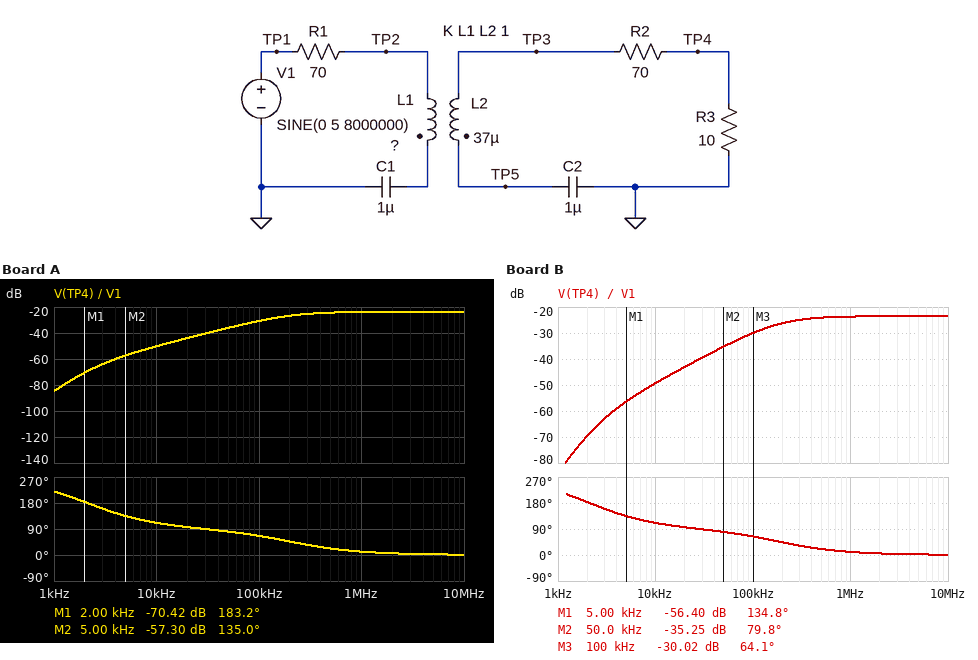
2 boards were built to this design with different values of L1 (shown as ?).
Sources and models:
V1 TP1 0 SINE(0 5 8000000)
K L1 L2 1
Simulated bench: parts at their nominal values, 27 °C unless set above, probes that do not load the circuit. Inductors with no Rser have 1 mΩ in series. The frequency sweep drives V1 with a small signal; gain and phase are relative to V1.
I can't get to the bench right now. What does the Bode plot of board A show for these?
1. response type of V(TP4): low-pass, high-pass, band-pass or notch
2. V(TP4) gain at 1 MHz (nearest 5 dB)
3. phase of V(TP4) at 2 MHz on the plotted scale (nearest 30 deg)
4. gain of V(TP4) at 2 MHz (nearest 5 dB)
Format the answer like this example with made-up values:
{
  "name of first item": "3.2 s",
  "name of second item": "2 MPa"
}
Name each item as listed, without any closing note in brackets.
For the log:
{
  "response type of V(TP4): low-pass, high-pass, band-pass or notch": "high-pass",
  "V(TP4) gain at 1 MHz": "-25 dB",
  "phase of V(TP4) at 2 MHz on the plotted scale": "0 deg",
  "gain of V(TP4) at 2 MHz": "-25 dB"
}
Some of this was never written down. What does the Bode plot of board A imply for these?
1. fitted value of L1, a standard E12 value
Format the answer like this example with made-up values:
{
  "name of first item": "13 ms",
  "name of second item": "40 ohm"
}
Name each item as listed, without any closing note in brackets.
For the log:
{
  "fitted value of L1, a standard E12 value": "22 µH"
}
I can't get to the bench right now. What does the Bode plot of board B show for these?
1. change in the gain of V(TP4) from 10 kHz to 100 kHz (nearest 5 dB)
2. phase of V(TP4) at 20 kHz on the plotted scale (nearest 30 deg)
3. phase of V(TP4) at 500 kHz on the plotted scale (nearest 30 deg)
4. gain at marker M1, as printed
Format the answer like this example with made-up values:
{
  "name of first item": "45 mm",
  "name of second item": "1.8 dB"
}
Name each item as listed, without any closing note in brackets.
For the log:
{
  "change in the gain of V(TP4) from 10 kHz to 100 kHz": "20 dB",
  "phase of V(TP4) at 20 kHz on the plotted scale": "90 deg",
  "phase of V(TP4) at 500 kHz on the plotted scale": "30 deg",
  "gain at marker M1, as printed": "-56.40 dB"
}
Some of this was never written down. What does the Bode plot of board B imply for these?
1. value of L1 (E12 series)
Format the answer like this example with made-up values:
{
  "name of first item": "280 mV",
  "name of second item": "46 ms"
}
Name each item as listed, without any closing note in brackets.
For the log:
{
  "value of L1": "27 µH"
}
